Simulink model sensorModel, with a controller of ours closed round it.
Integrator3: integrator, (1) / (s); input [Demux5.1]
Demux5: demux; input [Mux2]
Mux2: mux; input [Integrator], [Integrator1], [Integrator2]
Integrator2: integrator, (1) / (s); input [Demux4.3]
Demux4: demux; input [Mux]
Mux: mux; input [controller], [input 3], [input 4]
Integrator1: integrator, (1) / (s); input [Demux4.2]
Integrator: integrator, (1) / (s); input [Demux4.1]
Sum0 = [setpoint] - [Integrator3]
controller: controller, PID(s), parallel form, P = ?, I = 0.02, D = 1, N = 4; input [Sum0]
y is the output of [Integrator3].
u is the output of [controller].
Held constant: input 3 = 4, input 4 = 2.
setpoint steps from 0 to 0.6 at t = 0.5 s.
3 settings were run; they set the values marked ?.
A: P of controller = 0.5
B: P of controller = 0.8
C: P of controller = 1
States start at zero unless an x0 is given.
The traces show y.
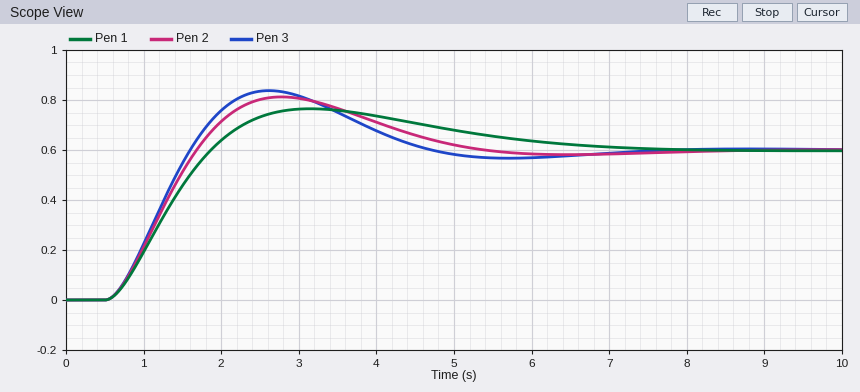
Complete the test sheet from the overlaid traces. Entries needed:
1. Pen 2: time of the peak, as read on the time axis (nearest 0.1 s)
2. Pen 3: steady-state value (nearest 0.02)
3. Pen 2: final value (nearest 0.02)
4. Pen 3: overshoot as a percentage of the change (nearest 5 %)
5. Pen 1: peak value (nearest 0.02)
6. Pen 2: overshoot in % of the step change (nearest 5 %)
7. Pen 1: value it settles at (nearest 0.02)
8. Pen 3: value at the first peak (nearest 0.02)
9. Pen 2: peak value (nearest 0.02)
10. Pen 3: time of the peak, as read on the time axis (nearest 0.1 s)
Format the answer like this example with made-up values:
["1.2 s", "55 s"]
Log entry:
["2.8 s", "0.60", "0.60", "40 %", "0.76", "35 %", "0.60", "0.84", "0.82", "2.6 s"]
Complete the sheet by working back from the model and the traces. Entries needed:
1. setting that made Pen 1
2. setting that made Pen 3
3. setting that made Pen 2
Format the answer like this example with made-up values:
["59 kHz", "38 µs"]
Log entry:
["A", "C", "B"]
